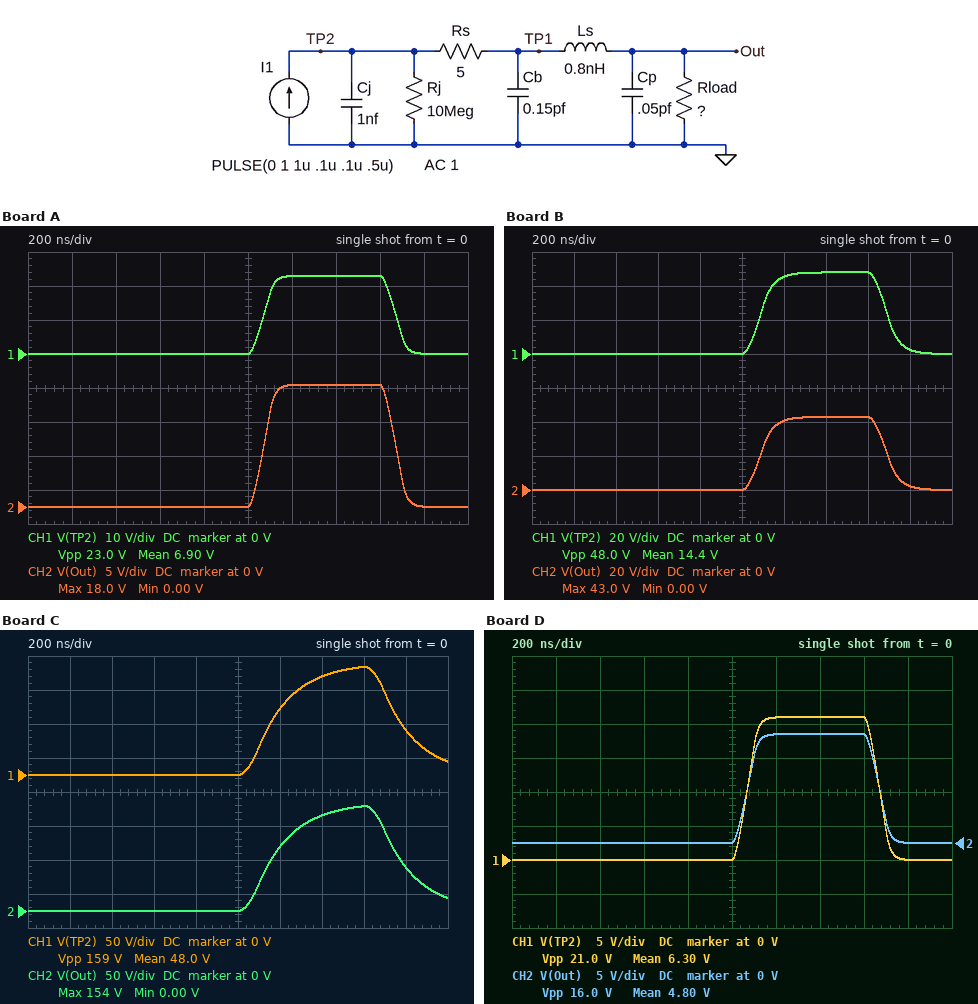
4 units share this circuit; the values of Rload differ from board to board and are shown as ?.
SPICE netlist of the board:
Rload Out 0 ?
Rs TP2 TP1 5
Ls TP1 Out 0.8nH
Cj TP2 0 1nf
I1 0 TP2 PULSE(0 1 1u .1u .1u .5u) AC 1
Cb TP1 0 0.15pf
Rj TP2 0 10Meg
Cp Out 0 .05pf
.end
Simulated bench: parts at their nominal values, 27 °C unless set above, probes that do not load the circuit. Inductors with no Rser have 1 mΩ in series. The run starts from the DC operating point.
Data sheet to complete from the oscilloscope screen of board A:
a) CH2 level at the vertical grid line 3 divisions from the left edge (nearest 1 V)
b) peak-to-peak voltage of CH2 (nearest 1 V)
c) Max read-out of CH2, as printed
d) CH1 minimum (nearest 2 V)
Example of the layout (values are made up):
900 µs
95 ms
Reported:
0 V
18 V
18.0 V
0 V
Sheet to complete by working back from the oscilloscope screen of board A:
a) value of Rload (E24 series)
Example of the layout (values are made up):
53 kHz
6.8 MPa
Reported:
18 Ω
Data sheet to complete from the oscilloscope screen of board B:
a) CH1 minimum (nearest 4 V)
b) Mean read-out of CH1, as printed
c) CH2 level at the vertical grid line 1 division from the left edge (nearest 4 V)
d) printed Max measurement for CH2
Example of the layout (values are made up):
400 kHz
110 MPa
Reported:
0 V
14.4 V
0 V
43.0 V
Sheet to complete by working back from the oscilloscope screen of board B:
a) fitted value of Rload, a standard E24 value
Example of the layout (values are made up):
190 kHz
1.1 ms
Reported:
43 Ω
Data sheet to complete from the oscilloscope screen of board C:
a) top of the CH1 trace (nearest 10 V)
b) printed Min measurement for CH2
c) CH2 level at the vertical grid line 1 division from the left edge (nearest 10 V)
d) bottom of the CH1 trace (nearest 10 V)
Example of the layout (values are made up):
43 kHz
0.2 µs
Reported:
160 V
0.00 V
0 V
0 V
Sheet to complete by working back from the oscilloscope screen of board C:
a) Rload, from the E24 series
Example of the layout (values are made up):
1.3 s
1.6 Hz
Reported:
160 Ω
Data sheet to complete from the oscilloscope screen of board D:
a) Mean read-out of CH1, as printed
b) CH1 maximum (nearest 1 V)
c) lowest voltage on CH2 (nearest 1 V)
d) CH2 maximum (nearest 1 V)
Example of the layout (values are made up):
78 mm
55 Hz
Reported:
6.30 V
21 V
0 V
16 V
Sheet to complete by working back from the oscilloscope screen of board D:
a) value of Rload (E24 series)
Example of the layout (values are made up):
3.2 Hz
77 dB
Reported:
16 Ω
